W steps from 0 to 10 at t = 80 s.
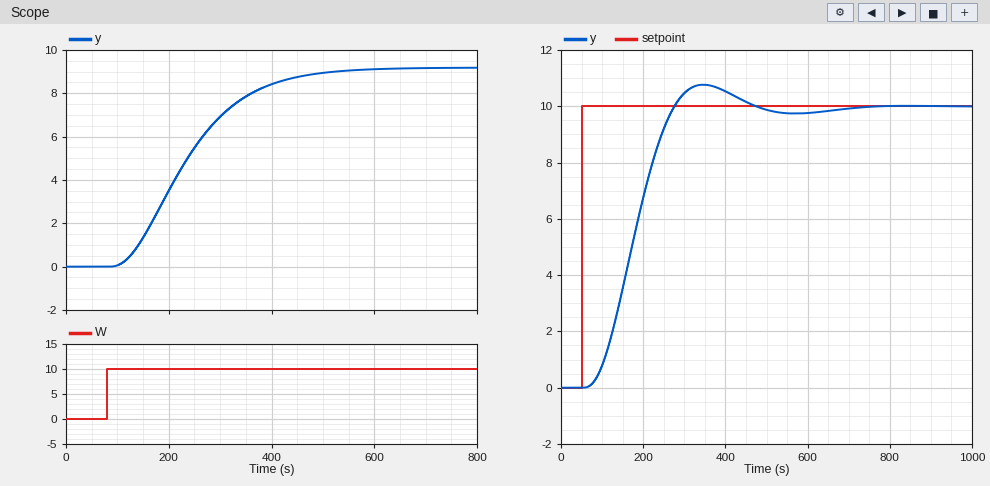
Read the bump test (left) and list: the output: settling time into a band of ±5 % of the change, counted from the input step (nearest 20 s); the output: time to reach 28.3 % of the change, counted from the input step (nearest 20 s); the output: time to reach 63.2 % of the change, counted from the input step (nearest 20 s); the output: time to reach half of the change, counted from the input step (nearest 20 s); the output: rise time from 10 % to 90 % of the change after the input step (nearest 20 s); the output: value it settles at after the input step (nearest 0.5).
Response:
360 s
100 s
180 s
140 s
240 s
9.0
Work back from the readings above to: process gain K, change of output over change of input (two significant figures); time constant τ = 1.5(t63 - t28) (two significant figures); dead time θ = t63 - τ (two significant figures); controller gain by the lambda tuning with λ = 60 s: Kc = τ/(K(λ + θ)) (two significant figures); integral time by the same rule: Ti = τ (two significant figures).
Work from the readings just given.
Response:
0.90
120 s
60 s
1.1
120 s
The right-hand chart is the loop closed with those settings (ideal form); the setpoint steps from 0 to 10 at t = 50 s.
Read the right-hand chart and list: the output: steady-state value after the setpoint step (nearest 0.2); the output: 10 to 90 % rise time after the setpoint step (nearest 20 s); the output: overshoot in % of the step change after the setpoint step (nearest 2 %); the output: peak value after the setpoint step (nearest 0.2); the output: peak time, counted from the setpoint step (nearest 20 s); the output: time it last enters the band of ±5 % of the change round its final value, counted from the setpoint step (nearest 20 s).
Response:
10.0
140 s
8 %
10.8
300 s
360 s
